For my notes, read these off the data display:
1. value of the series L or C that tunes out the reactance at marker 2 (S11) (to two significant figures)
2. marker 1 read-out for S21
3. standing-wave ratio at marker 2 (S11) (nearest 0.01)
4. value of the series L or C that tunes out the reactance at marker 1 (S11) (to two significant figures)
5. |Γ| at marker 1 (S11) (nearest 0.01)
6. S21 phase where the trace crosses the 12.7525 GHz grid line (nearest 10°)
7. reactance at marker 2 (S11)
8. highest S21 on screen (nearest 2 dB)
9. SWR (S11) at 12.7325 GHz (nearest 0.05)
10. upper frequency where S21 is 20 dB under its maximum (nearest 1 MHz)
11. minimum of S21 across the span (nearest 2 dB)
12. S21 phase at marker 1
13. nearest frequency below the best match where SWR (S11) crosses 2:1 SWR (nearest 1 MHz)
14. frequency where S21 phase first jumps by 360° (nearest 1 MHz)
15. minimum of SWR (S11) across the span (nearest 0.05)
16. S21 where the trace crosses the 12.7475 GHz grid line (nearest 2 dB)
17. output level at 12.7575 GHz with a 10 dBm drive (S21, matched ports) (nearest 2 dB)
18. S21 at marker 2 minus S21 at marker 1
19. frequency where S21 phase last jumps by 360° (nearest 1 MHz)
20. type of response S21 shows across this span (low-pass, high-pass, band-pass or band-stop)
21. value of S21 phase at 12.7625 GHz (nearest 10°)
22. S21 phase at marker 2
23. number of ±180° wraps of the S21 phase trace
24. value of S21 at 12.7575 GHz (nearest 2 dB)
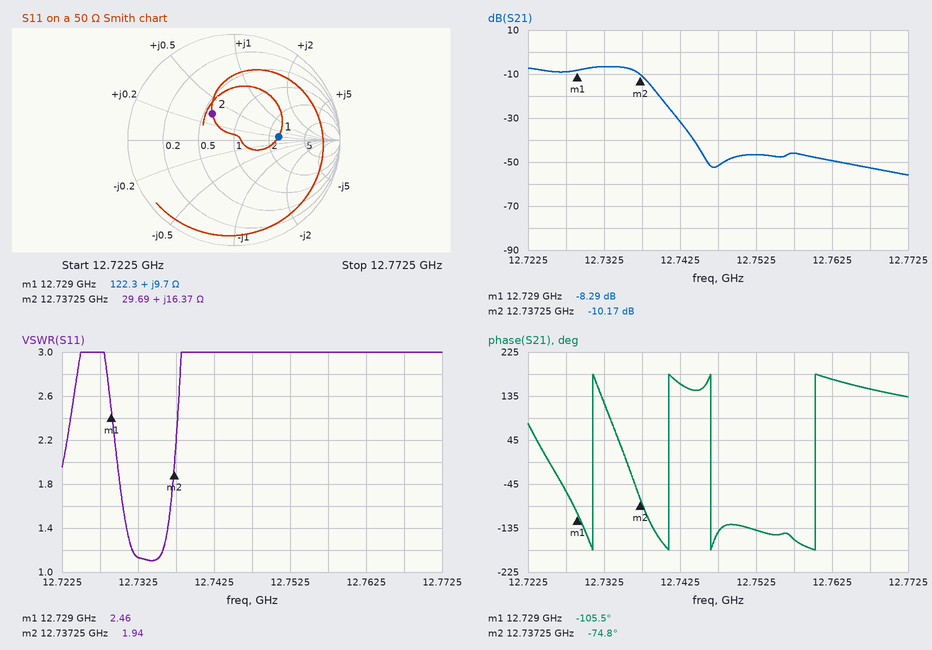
760 fF
-8.29 dB
1.94
1.3 pF
0.42
-140°
+16.37 Ω
-6 dB
1.15
12.741 GHz
-56 dB
-105.5°
12.730 GHz
12.731 GHz
1.10
-52 dB
-36 dBm
-1.88 dB
12.760 GHz
low-pass
170°
-74.8°
4
-46 dB
